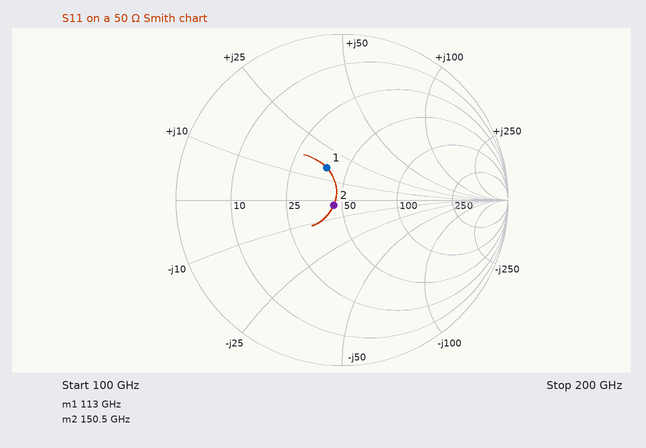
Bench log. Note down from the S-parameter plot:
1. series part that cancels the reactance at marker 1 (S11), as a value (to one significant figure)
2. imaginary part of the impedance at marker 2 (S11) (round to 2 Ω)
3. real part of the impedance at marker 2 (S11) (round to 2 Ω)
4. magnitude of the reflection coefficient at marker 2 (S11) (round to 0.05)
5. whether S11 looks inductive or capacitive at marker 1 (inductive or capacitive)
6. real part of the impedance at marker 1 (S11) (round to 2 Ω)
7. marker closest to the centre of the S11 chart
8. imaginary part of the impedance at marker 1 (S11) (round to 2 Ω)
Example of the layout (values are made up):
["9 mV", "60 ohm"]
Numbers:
["90 fF", "-2 Ω", "46 Ω", "0.05", "inductive", "38 Ω", "marker 2", "+16 Ω"]
